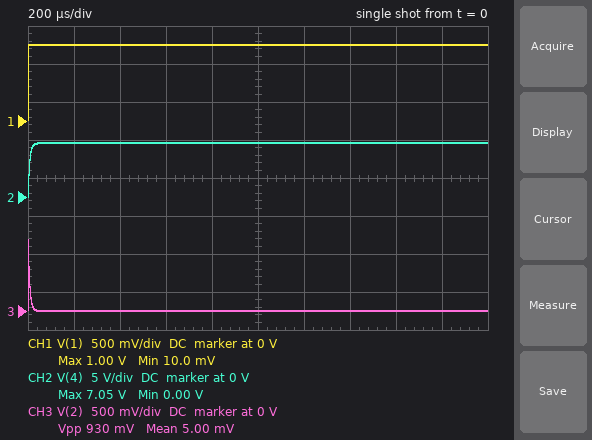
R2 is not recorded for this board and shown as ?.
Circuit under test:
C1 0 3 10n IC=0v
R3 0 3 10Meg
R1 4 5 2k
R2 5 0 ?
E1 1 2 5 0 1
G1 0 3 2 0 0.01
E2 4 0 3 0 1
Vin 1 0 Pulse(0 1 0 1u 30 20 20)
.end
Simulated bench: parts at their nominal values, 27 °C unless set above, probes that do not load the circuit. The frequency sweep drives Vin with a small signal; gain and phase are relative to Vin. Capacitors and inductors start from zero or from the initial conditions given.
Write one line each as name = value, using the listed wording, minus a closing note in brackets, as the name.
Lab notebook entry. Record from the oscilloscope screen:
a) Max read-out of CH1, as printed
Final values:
Max read-out of CH1, as printed = 1.00 V
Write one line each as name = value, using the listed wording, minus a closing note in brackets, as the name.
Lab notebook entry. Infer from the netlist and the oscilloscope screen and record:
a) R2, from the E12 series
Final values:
R2, from the E12 series = 330 Ω
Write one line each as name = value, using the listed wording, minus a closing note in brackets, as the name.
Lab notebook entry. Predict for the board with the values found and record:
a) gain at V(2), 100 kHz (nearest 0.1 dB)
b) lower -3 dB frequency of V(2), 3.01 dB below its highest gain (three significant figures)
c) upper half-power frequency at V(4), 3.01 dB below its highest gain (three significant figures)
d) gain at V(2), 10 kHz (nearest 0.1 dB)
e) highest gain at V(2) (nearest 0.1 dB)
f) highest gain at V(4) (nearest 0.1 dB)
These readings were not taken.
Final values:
gain at V(2), 100 kHz = -0.2 dB
lower -3 dB frequency of V(2), 3.01 dB below its highest gain = 22.5 kHz
upper half-power frequency at V(4), 3.01 dB below its highest gain = 22.5 kHz
gain at V(2), 10 kHz = -7.8 dB
highest gain at V(2) = 0 dB
highest gain at V(4) = 17.0 dB
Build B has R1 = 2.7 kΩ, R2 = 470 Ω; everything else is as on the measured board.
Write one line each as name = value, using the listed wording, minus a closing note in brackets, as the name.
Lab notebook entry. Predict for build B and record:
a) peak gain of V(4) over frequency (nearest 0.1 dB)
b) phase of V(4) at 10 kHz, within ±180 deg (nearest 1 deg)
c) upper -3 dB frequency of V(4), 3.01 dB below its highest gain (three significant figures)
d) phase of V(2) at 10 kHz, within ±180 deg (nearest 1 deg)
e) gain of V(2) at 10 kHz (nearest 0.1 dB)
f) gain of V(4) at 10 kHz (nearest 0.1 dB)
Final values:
peak gain of V(4) over frequency = 16.6 dB
phase of V(4) at 10 kHz, within ±180 deg = -23 deg
upper -3 dB frequency of V(4), 3.01 dB below its highest gain = 23.6 kHz
phase of V(2) at 10 kHz, within ±180 deg = 67 deg
gain of V(2) at 10 kHz = -8.2 dB
gain of V(4) at 10 kHz = 15.9 dB
